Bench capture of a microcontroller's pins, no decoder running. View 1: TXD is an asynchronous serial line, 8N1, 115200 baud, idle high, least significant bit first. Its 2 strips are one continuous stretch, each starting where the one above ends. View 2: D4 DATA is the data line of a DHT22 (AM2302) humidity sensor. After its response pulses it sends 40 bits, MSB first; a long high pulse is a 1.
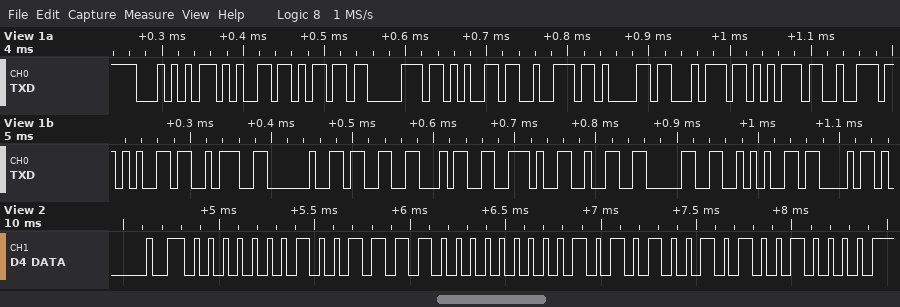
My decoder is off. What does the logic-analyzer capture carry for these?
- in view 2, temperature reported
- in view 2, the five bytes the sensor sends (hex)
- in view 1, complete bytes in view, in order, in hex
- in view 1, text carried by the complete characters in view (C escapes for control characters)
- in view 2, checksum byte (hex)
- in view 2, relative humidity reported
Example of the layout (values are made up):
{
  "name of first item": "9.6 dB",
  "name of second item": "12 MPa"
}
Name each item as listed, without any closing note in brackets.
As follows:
{
  "in view 2, temperature reported": "33.8 °C",
  "in view 2, the five bytes the sensor sends": "01 3C 01 52 90",
  "in view 1, complete bytes in view, in order, in hex": "54 65 6D 70 65 72 61 74 75 72 65 3A 20 33 34 2E 32 30 2A 43",
  "in view 1, text carried by the complete characters in view": "\"Temperature: 34.20*C\"",
  "in view 2, checksum byte": "0x90",
  "in view 2, relative humidity reported": "31.6 %"
}
